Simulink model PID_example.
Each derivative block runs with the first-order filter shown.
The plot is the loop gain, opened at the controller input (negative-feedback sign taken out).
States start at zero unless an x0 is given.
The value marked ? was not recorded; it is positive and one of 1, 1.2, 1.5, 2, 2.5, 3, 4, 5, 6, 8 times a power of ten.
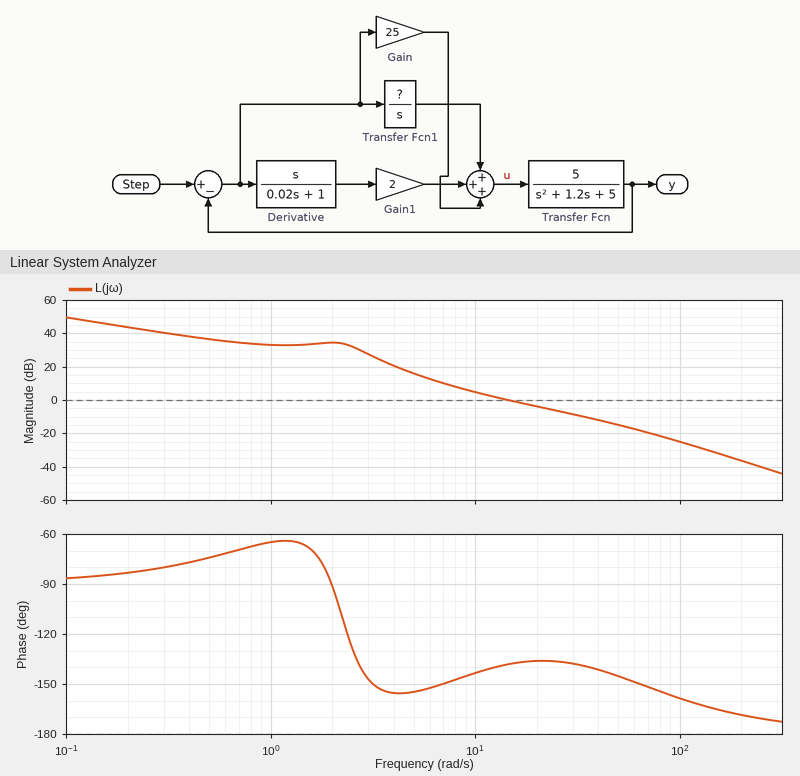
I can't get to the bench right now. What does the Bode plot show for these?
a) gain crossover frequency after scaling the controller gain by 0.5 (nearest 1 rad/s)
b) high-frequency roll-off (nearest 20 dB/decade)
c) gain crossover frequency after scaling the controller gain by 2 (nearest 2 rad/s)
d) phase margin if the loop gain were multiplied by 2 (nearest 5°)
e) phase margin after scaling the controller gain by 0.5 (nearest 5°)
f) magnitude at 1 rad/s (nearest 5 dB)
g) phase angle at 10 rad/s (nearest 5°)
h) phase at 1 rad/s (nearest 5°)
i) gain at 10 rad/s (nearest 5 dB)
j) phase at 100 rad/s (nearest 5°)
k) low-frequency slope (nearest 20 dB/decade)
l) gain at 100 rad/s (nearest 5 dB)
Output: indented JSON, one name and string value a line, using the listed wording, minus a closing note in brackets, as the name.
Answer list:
{
  "gain crossover frequency after scaling the controller gain by 0.5": "9 rad/s",
  "high-frequency roll-off": "-40 dB/decade",
  "gain crossover frequency after scaling the controller gain by 2": "24 rad/s",
  "phase margin if the loop gain were multiplied by 2": "45°",
  "phase margin after scaling the controller gain by 0.5": "35°",
  "magnitude at 1 rad/s": "35 dB",
  "phase angle at 10 rad/s": "-145°",
  "phase at 1 rad/s": "-65°",
  "gain at 10 rad/s": "5 dB",
  "phase at 100 rad/s": "-160°",
  "low-frequency slope": "-20 dB/decade",
  "gain at 100 rad/s": "-25 dB"
}
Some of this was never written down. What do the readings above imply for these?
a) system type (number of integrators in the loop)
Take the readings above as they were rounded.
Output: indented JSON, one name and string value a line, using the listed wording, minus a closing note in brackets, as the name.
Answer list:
{
  "system type": "1"
}
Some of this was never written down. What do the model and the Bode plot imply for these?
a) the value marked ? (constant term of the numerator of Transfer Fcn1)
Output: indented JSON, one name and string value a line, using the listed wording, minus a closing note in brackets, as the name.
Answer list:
{
  "the value marked ?": "30"
}
